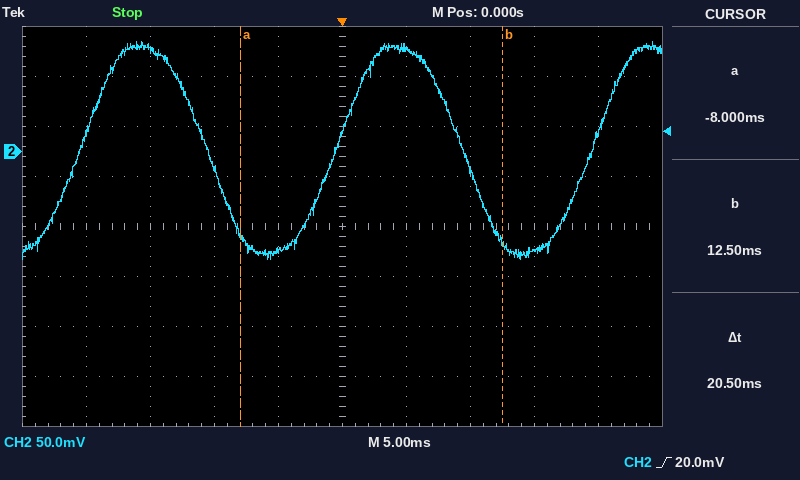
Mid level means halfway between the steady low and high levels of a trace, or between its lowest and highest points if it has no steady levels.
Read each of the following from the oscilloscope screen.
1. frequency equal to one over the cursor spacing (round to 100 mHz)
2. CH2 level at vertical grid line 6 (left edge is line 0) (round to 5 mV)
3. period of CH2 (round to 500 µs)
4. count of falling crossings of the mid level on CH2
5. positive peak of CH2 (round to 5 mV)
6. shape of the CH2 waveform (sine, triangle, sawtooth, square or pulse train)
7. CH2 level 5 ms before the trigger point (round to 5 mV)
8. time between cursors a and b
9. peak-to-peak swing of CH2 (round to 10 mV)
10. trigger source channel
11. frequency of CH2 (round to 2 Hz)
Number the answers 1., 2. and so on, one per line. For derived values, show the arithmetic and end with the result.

1. 1 / 20.5 ms ≈ 48.8 Hz
2. 105 mV
3. 20.0 ms
4. 2
5. 110 mV
6. sine
7. -100 mV
8. 20.5 ms
9. 220 mV
10. CH2
11. 1 / 20.0 ms ≈ 50 Hz
